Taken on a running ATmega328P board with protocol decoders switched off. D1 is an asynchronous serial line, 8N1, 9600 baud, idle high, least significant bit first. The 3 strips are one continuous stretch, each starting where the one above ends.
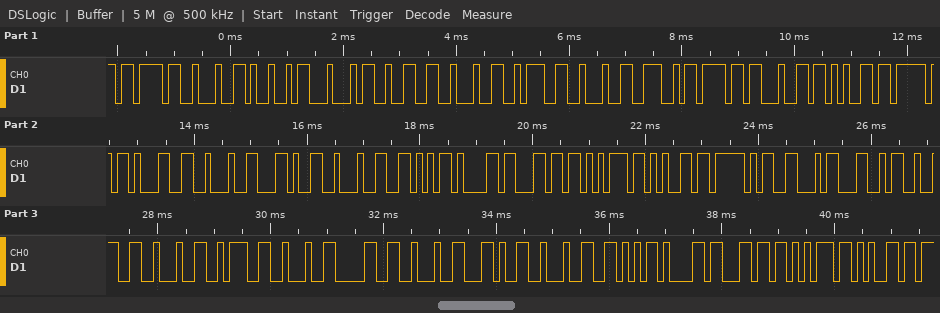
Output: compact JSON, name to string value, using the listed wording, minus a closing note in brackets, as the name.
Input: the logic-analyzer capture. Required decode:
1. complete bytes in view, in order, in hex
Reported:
{"complete bytes in view, in order, in hex": "0x7B 0x22 0x49 0x44 0x32 0x22 0x3A 0x22 0x4E 0x6F 0x64 0x65 0x5F 0x31 0x22 0x2C 0x22 0x56 0x61 0x6C 0x75 0x65 0x5F 0x46 0x4C 0x32 0x22 0x3A 0x22 0x30 0x22 0x2C 0x22 0x56 0x61 0x6C 0x75 0x65"}
